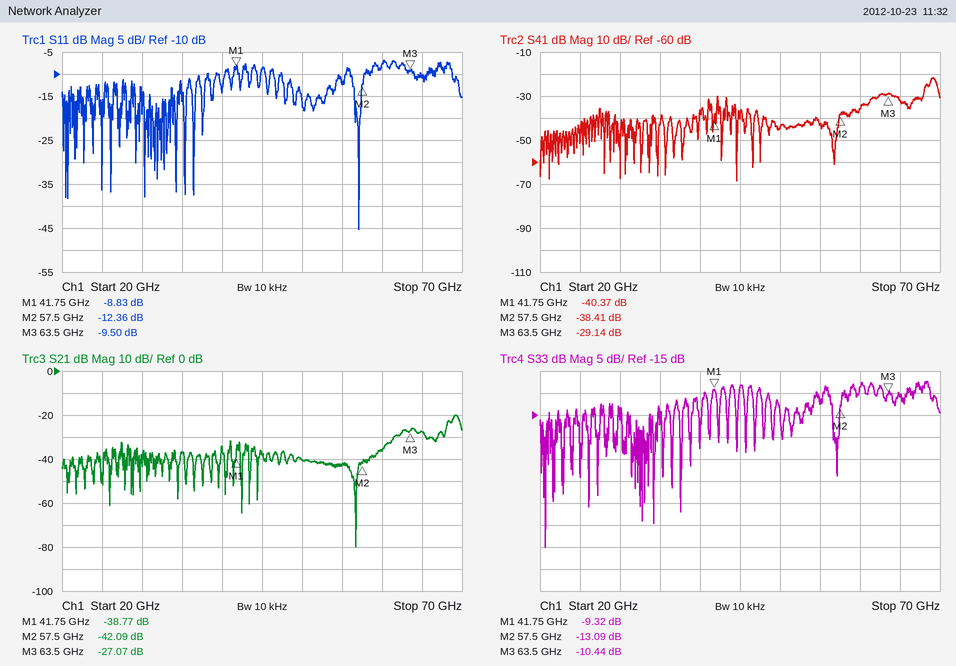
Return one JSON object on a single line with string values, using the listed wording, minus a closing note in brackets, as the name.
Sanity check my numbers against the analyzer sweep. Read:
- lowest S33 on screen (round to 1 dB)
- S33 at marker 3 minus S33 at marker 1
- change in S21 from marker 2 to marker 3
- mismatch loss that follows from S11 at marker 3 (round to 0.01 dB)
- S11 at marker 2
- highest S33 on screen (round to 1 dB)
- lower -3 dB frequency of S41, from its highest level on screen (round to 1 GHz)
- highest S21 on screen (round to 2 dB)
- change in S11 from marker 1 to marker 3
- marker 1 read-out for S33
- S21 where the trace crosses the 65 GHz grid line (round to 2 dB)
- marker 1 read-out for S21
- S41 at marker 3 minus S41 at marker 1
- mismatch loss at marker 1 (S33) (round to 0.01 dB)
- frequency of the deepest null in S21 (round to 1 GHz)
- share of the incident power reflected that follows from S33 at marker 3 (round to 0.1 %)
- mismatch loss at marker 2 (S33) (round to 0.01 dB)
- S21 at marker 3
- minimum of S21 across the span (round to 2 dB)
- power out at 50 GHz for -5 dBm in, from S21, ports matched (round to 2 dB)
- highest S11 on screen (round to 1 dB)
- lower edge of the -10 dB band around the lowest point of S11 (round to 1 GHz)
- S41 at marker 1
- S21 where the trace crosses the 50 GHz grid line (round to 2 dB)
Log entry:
{"lowest S33 on screen": "-45 dB", "S33 at marker 3 minus S33 at marker 1": "-1.12 dB", "change in S21 from marker 2 to marker 3": "15.02 dB", "mismatch loss that follows from S11 at marker 3": "0.52 dB", "S11 at marker 2": "-12.36 dB", "highest S33 on screen": "-7 dB", "lower -3 dB frequency of S41, from its highest level on screen": "69 GHz", "highest S21 on screen": "-20 dB", "change in S11 from marker 1 to marker 3": "-0.67 dB", "marker 1 read-out for S33": "-9.32 dB", "S21 where the trace crosses the 65 GHz grid line": "-28 dB", "marker 1 read-out for S21": "-38.77 dB", "S41 at marker 3 minus S41 at marker 1": "11.23 dB", "mismatch loss at marker 1 (S33)": "0.54 dB", "frequency of the deepest null in S21": "57 GHz", "share of the incident power reflected that follows from S33 at marker 3": "9.0 %", "mismatch loss at marker 2 (S33)": "0.22 dB", "S21 at marker 3": "-27.07 dB", "minimum of S21 across the span": "-80 dB", "power out at 50 GHz for -5 dBm in, from S21, ports matched": "-46 dBm", "highest S11 on screen": "-7 dB", "lower edge of the -10 dB band around the lowest point of S11": "56 GHz", "S41 at marker 1": "-40.37 dB", "S21 where the trace crosses the 50 GHz grid line": "-40 dB"}
